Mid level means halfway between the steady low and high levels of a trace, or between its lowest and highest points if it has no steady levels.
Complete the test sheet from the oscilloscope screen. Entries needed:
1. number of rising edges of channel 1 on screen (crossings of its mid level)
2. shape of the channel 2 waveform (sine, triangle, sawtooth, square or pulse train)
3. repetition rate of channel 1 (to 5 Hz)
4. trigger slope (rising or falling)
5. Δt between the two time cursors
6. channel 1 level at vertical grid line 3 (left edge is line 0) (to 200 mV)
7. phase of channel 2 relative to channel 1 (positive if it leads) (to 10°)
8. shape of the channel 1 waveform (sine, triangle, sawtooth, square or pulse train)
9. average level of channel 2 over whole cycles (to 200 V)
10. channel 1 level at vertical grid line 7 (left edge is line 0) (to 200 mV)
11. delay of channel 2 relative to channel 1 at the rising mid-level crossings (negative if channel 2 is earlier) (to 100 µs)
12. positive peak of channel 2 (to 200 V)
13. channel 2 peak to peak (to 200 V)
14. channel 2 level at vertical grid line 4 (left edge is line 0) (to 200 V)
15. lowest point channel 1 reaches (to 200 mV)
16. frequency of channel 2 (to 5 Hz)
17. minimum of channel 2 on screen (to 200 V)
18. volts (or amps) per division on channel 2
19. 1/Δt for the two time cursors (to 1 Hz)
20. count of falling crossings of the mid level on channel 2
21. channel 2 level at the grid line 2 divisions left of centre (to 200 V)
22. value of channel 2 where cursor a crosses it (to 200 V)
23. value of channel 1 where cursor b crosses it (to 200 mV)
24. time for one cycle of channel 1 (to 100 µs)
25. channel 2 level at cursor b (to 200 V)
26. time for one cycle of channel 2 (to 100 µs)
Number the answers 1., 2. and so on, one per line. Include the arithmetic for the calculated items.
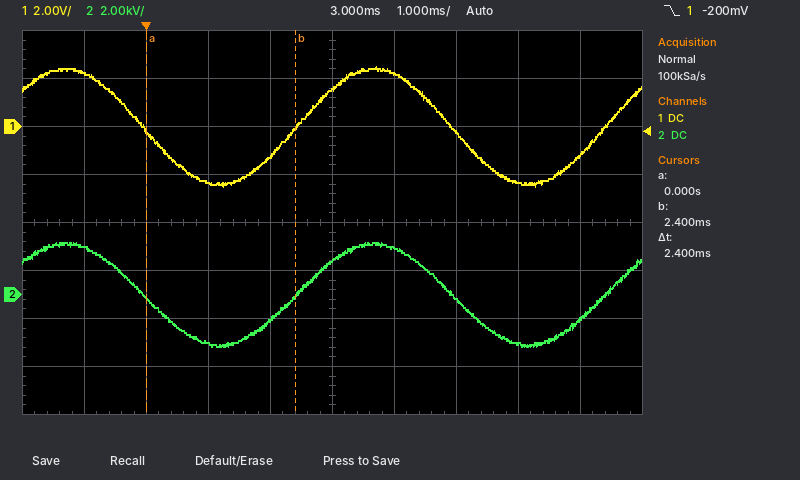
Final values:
1. 2
2. sine
3. 1 / 5.0 ms ≈ 200 Hz
4. falling
5. 2.4 ms
6. -2.4 V
7. −360° × (0.0 ms) / 5.0 ms ≈ 0°
8. sine
9. (2.2 kV + (-2.2 kV)) / 2 ≈ 0.0 kV
10. -200 mV
11. 0.0 ms
12. 2.2 kV
13. 2.2 kV − (-2.2 kV) = 4.4 kV
14. -1.0 kV
15. -2.4 V
16. 1 / 5.0 ms ≈ 200 Hz
17. -2.2 kV
18. 2 kV
19. 1 / 2.4 ms ≈ 417 Hz
20. 2
21. -2.0 kV
22. -200 V
23. 0.0 V
24. 5.0 ms
25. 0.0 kV
26. 5.0 ms
